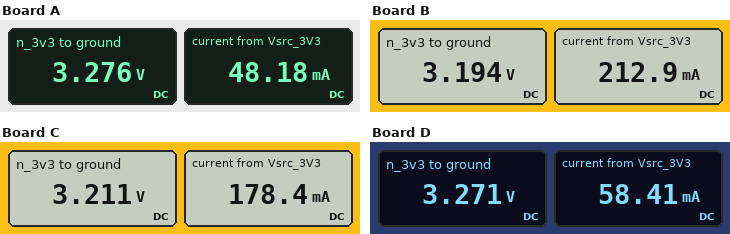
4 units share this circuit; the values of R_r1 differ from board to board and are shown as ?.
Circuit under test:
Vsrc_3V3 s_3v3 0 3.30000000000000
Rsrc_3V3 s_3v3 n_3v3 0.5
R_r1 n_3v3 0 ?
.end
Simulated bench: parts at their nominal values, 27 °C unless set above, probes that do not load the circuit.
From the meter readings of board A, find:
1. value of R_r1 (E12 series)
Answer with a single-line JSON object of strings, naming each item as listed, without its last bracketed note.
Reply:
{"value of R_r1": "68 Ω"}
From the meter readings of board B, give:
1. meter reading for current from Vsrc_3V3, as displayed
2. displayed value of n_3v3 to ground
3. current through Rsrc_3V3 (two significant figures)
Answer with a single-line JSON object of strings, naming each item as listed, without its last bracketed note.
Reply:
{"meter reading for current from Vsrc_3V3, as displayed": "212.9 mA", "displayed value of n_3v3 to ground": "3.194 V", "current through Rsrc_3V3": "210 mA"}
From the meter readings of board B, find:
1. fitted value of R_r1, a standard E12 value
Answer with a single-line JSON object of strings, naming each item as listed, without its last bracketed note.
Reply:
{"fitted value of R_r1, a standard E12 value": "15 Ω"}
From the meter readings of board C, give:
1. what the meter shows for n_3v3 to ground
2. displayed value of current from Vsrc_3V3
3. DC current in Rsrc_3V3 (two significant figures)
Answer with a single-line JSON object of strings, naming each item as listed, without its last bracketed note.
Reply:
{"what the meter shows for n_3v3 to ground": "3.211 V", "displayed value of current from Vsrc_3V3": "178.4 mA", "DC current in Rsrc_3V3": "180 mA"}
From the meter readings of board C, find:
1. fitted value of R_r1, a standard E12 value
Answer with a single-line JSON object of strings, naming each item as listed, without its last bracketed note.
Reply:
{"fitted value of R_r1, a standard E12 value": "18 Ω"}
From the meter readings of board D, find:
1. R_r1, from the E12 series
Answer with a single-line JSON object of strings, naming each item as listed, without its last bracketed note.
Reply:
{"R_r1, from the E12 series": "56 Ω"}
